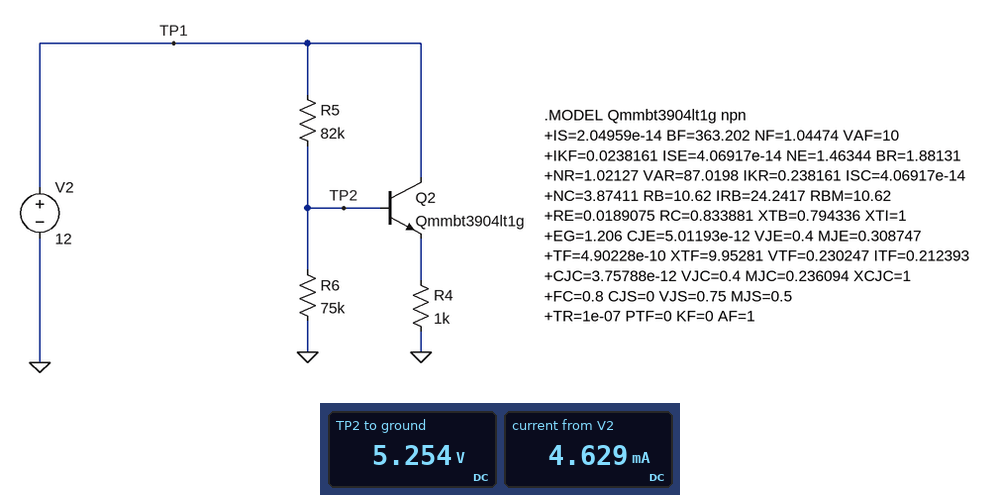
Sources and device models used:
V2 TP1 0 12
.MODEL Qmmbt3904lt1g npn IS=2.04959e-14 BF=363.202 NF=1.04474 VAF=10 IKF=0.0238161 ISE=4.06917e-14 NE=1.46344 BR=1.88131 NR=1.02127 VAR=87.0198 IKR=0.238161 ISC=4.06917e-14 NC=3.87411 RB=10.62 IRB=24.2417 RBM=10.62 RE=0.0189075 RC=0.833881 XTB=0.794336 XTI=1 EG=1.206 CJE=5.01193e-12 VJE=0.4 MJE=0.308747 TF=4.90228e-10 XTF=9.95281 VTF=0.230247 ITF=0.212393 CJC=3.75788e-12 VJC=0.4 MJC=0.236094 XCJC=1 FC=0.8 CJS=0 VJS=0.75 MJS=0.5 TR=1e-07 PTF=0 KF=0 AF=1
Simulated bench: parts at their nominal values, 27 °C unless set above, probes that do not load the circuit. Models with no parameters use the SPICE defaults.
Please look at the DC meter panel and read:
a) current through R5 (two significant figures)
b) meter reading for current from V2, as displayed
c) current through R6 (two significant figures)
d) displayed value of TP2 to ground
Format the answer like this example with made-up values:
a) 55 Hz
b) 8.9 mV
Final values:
a) 82 µA
b) 4.629 mA
c) 70 µA
d) 5.254 V
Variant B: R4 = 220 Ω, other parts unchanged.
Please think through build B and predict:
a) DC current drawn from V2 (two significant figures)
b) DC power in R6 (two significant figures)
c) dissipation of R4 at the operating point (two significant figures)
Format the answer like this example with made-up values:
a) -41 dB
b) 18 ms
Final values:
a) 15 mA
b) 220 µW
c) 51 mW
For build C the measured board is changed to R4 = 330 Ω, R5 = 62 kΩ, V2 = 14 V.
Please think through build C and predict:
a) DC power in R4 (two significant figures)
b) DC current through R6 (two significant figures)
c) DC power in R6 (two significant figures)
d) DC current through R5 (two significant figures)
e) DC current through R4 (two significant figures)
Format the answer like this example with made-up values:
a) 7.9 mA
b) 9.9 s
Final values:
a) 88 mW
b) 82 µA
c) 500 µW
d) 130 µA
e) 16 mA
